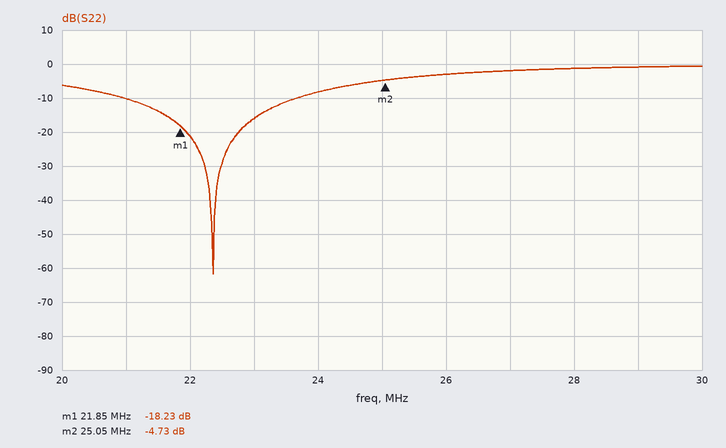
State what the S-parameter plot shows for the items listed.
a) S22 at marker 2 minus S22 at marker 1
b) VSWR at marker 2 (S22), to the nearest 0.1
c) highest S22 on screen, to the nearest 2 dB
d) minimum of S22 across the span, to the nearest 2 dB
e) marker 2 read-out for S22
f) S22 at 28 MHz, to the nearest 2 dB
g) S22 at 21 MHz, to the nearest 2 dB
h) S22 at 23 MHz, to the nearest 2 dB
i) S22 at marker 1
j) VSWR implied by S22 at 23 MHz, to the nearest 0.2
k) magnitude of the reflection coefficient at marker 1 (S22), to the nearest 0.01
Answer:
13.50 dB
3.8
0 dB
-62 dB
-4.73 dB
-2 dB
-10 dB
-16 dB
-18.23 dB
1.4
0.12
